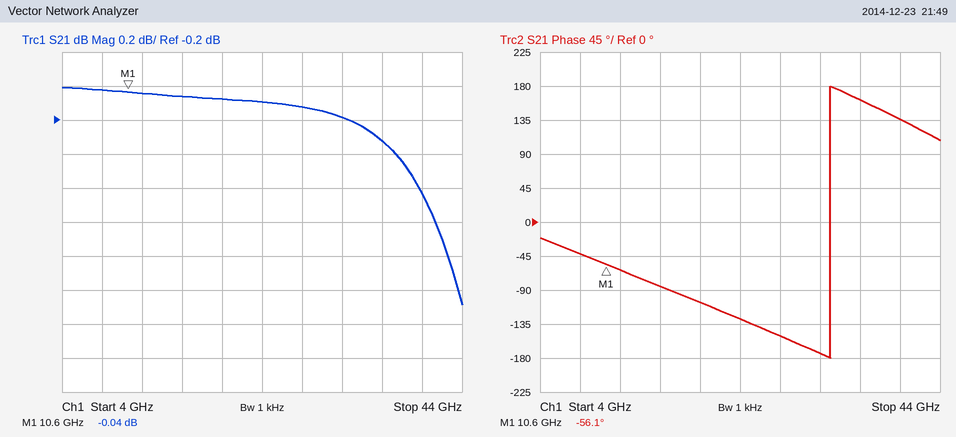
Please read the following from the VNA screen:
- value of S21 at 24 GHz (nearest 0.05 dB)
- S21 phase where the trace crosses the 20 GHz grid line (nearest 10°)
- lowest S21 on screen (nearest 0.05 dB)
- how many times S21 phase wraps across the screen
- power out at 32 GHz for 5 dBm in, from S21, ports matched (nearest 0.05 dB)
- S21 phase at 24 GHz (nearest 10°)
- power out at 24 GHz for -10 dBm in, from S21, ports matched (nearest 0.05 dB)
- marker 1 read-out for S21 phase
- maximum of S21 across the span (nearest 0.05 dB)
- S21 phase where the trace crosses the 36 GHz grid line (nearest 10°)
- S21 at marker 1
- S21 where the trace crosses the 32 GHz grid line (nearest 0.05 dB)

-0.10 dB
-110°
-1.30 dB
1
4.80 dBm
-130°
-10.10 dBm
-56.1°
0.00 dB
160°
-0.04 dB
-0.20 dB
